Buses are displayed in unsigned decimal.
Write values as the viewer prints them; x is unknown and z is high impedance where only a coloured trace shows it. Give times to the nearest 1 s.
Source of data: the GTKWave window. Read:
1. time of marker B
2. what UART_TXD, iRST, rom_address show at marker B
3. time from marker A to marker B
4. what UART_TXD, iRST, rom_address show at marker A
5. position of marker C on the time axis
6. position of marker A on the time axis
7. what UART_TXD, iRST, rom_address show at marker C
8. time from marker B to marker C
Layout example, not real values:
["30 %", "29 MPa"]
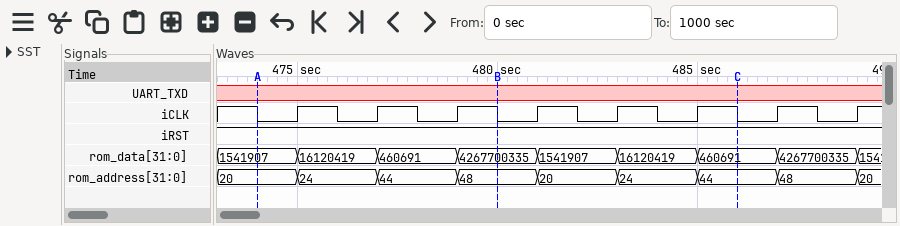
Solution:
["480 s", "UART_TXD=x, iRST=1, rom_address=48", "6 s", "UART_TXD=x, iRST=1, rom_address=20", "486 s", "474 s", "UART_TXD=x, iRST=1, rom_address=44", "6 s"]
